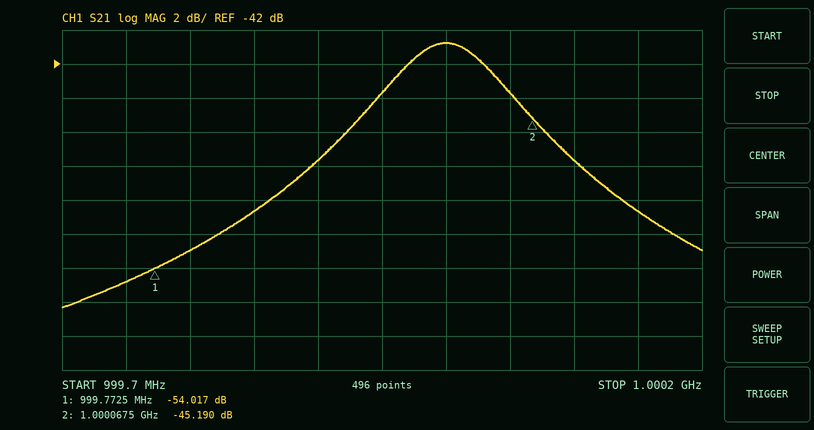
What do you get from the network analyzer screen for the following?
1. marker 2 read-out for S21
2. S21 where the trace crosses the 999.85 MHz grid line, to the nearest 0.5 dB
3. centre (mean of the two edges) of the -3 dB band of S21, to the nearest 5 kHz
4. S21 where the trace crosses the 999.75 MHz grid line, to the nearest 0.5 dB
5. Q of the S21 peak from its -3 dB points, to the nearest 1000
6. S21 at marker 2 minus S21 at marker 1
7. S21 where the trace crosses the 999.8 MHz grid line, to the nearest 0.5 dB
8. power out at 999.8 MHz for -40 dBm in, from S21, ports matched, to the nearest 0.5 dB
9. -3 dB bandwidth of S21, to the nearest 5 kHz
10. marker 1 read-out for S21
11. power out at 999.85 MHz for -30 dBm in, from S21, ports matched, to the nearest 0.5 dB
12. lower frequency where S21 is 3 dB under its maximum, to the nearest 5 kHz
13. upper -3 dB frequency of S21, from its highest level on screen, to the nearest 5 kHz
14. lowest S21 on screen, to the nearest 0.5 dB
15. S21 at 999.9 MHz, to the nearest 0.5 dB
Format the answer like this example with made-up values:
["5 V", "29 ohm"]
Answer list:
["-45.190 dB", "-50.5 dB", "1.000000 GHz", "-55.0 dB", "10000", "8.827 dB", "-53.0 dB", "-93.0 dBm", "100 kHz", "-54.017 dB", "-80.5 dBm", "999.950 MHz", "1.000050 GHz", "-56.5 dB", "-47.5 dB"]
